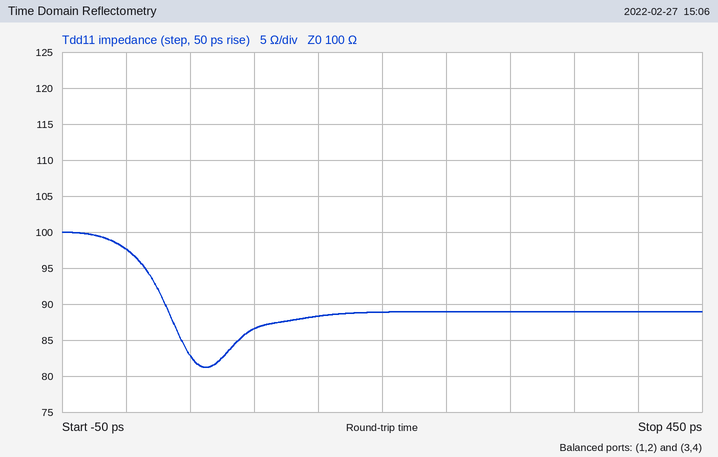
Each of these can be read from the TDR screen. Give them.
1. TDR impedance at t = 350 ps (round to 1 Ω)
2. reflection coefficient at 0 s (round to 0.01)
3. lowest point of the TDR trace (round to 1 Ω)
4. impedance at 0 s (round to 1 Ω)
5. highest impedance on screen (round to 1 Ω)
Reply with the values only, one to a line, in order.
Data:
89 Ω
-0.01
81 Ω
98 Ω
100 Ω
